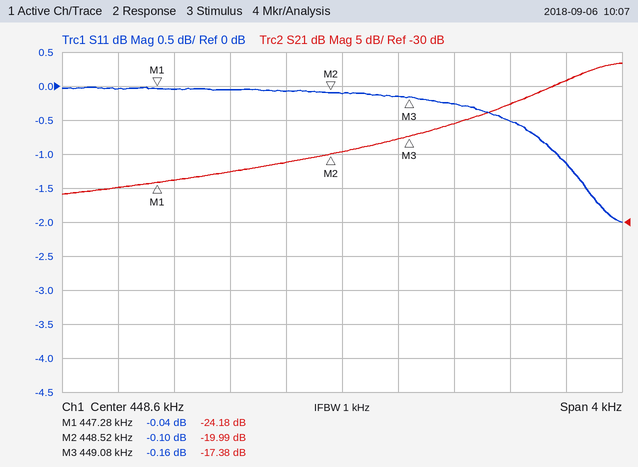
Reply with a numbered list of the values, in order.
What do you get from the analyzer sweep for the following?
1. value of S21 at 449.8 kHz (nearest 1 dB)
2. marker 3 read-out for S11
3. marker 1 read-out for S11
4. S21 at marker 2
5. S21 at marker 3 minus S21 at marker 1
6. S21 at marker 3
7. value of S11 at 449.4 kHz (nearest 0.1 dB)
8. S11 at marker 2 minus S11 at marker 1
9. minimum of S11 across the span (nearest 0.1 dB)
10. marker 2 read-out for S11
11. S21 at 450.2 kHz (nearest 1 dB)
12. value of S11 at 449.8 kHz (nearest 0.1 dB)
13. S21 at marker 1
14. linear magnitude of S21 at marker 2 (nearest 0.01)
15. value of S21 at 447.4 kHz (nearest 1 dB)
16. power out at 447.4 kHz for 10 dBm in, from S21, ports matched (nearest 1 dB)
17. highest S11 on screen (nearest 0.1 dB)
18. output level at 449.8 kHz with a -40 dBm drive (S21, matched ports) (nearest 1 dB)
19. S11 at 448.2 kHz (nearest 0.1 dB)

1. -13 dB
2. -0.16 dB
3. -0.04 dB
4. -19.99 dB
5. 6.80 dB
6. -17.38 dB
7. -0.3 dB
8. -0.06 dB
9. -2.0 dB
10. -0.10 dB
11. -9 dB
12. -0.5 dB
13. -24.18 dB
14. 0.10
15. -24 dB
16. -14 dBm
17. 0.0 dB
18. -53 dBm
19. -0.1 dB
